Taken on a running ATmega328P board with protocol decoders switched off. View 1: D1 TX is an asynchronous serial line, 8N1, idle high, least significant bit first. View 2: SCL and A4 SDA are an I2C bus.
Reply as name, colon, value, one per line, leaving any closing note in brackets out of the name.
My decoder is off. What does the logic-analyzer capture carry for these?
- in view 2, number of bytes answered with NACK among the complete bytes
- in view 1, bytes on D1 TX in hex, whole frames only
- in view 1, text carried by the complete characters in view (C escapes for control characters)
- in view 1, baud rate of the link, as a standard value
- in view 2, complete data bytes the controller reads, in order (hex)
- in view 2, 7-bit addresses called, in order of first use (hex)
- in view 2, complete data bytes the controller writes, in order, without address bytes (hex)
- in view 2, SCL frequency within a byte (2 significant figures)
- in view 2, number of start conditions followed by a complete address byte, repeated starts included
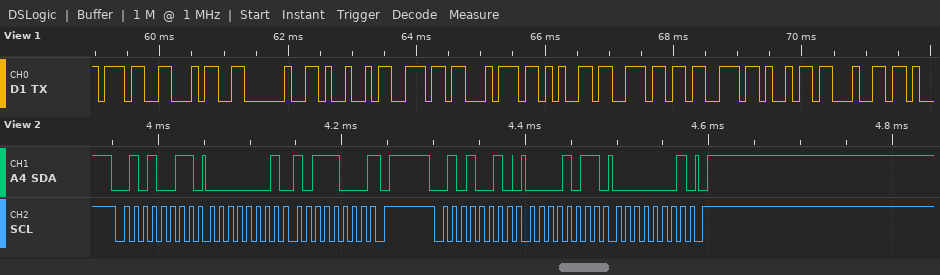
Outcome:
in view 2, number of bytes answered with NACK among the complete bytes: 1
in view 1, bytes on D1 TX in hex, whole frames only: 0x37 0x34 0x20 0x49 0x6E 0x74 0x65 0x6E 0x73 0x69 0x64
in view 1, text carried by the complete characters in view: "74 Intensid"
in view 1, baud rate of the link, as a standard value: 9600 baud
in view 2, complete data bytes the controller reads, in order: 01 B8
in view 2, 7-bit addresses called, in order of first use: 0x29
in view 2, complete data bytes the controller writes, in order, without address bytes: 0B 01
in view 2, SCL frequency within a byte: 100 kHz
in view 2, number of start conditions followed by a complete address byte, repeated starts included: 2
